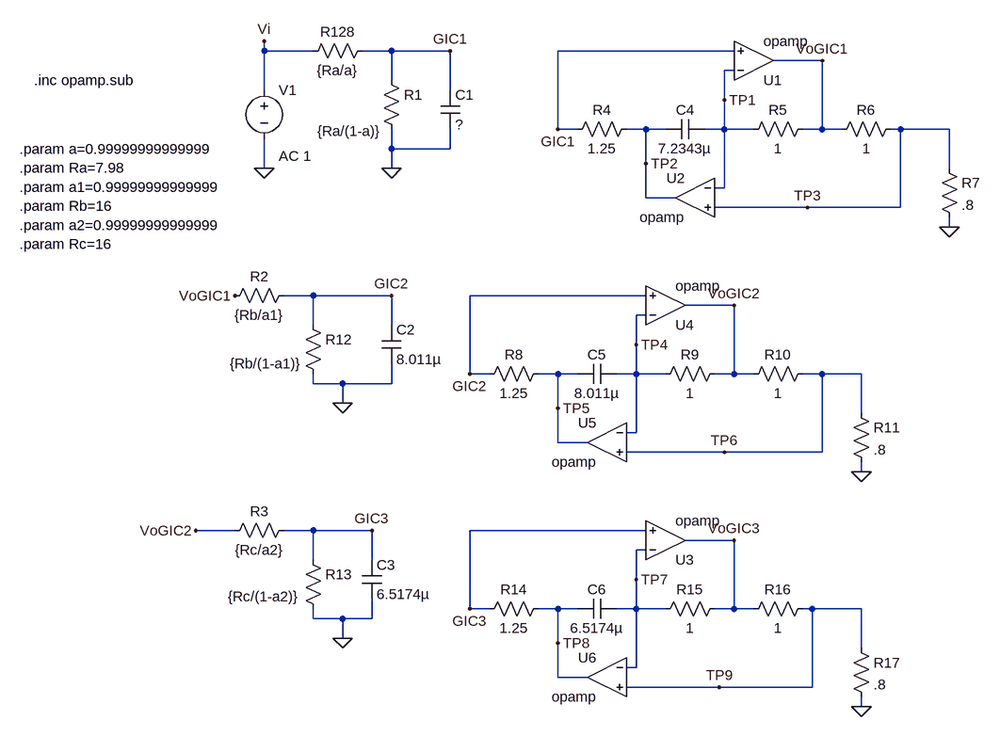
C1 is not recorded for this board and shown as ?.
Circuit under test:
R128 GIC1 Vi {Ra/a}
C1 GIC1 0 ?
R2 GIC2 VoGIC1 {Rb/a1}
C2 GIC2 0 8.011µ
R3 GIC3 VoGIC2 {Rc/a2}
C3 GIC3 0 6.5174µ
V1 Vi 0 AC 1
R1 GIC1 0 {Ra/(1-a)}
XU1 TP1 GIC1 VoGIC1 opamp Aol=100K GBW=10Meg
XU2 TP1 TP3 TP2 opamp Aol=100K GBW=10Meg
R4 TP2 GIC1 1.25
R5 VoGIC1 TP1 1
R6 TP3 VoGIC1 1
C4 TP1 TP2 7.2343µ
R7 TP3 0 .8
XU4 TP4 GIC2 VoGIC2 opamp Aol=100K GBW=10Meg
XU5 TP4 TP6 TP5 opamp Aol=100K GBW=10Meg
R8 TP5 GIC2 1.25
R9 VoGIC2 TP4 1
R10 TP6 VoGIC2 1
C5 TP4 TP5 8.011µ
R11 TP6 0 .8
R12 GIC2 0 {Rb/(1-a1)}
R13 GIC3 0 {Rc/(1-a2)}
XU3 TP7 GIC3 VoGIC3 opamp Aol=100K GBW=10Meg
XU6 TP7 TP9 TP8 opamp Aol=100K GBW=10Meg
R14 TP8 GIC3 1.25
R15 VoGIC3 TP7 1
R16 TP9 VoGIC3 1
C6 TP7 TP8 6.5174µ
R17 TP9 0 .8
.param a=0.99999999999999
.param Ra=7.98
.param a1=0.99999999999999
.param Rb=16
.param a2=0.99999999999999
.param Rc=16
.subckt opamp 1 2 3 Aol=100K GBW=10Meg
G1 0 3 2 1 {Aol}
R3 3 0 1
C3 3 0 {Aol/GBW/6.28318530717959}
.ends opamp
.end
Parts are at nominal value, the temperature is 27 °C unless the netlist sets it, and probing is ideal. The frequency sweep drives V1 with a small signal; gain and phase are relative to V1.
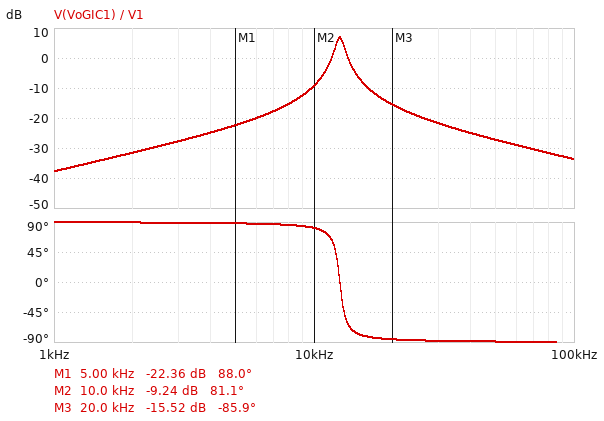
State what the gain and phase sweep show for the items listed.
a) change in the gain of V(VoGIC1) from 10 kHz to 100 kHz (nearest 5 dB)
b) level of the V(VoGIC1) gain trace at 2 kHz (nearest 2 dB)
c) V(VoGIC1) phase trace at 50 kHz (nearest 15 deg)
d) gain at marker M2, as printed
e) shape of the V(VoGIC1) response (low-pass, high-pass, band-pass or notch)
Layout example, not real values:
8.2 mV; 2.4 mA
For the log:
-25 dB; -32 dB; -90 deg; -9.24 dB; band-pass
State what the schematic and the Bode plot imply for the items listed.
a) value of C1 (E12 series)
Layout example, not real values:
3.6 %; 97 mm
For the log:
22 µF
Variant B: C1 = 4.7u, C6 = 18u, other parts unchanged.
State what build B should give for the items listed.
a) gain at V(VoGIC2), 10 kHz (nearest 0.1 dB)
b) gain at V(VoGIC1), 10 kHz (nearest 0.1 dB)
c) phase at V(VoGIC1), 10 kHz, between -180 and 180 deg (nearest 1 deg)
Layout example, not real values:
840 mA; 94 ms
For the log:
-37.0 dB; -16.6 dB; 86 deg
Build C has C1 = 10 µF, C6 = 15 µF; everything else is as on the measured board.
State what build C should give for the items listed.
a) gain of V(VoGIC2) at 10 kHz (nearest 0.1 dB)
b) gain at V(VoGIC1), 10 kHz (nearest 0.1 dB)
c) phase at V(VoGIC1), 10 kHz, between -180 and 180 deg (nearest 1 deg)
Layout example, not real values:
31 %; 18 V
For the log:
-35.3 dB; -14.9 dB; 85 deg
